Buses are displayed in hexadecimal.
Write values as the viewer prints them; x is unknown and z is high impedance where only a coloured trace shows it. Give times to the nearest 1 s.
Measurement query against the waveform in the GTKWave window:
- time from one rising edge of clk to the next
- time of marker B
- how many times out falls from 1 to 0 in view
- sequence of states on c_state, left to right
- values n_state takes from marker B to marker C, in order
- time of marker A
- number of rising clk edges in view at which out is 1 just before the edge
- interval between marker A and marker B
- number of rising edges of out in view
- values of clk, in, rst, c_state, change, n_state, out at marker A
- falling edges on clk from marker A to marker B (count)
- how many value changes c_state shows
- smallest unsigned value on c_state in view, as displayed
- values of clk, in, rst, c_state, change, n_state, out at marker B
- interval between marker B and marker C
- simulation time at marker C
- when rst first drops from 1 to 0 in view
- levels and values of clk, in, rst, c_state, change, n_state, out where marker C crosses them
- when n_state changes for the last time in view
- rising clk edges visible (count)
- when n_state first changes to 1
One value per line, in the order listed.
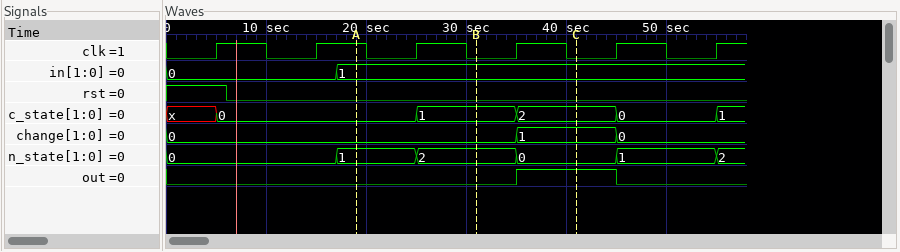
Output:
10 s
31 s
1
x, 0, 1, 2, 0, 1
2, 0
19 s
1
12 s
1
clk=1, in=1, rst=0, c_state=0, change=0, n_state=1, out=0
2
5
0
clk=0, in=1, rst=0, c_state=1, change=0, n_state=2, out=0
10 s
41 s
6 s
clk=0, in=1, rst=0, c_state=2, change=1, n_state=0, out=1
55 s
6
17 s
